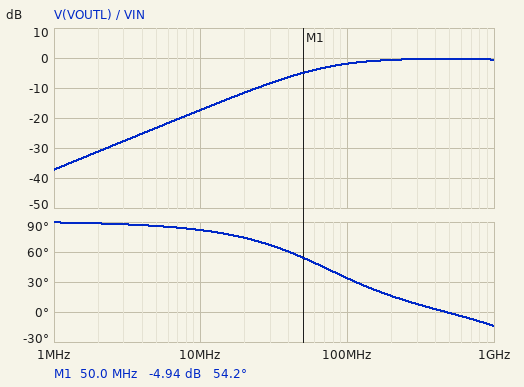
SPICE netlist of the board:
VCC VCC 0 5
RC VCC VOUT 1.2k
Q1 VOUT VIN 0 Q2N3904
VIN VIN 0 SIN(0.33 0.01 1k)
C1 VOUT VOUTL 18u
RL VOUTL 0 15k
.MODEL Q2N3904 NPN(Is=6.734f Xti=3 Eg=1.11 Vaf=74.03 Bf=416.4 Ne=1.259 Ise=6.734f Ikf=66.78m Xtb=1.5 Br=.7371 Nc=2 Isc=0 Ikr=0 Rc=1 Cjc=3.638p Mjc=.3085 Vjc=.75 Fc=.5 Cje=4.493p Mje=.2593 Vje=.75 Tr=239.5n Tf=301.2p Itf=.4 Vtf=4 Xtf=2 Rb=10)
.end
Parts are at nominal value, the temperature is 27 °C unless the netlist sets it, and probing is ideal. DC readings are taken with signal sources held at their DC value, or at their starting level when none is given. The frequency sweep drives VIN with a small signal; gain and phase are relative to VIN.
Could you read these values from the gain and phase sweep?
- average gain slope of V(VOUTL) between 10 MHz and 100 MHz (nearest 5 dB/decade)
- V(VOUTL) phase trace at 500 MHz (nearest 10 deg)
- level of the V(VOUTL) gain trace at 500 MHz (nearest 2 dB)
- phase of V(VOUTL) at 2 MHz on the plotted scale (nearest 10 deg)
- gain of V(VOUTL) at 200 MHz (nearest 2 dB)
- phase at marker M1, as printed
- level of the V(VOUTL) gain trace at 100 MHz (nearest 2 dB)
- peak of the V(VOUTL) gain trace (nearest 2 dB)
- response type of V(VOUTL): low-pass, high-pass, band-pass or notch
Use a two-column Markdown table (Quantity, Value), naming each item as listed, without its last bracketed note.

| Quantity | Value |
|---|---|
| average gain slope of V(VOUTL) between 10 MHz and 100 MHz | 15 dB/decade |
| V(VOUTL) phase trace at 500 MHz | 0 deg |
| level of the V(VOUTL) gain trace at 500 MHz | 0 dB |
| phase of V(VOUTL) at 2 MHz on the plotted scale | 90 deg |
| gain of V(VOUTL) at 200 MHz | 0 dB |
| phase at marker M1, as printed | 54.2 deg |
| level of the V(VOUTL) gain trace at 100 MHz | -2 dB |
| peak of the V(VOUTL) gain trace | 0 dB |
| response type of V(VOUTL): low-pass, high-pass, band-pass or notch | high-pass |
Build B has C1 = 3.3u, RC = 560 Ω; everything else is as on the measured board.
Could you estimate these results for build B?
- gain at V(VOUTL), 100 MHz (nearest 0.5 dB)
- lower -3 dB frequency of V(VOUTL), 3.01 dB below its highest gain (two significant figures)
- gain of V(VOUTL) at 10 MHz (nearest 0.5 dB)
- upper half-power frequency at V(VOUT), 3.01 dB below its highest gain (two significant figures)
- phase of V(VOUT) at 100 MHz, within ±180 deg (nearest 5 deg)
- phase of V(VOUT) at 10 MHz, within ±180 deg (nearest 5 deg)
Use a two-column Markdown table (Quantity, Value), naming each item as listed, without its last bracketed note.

| Quantity | Value |
|---|---|
| gain at V(VOUTL), 100 MHz | -5.0 dB |
| lower -3 dB frequency of V(VOUTL), 3.01 dB below its highest gain | 130 MHz |
| gain of V(VOUTL) at 10 MHz | -23.5 dB |
| upper half-power frequency at V(VOUT), 3.01 dB below its highest gain | 3.4 GHz |
| phase of V(VOUT) at 100 MHz, within ±180 deg | 55 deg |
| phase of V(VOUT) at 10 MHz, within ±180 deg | 85 deg |
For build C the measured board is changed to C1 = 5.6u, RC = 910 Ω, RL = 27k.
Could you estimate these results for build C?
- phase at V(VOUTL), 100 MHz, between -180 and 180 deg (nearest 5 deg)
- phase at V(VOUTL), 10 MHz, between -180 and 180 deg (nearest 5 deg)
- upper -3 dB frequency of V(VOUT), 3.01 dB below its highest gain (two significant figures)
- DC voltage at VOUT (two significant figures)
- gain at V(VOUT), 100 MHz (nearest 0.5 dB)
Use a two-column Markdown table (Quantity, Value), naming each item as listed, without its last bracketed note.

| Quantity | Value |
|---|---|
| phase at V(VOUTL), 100 MHz, between -180 and 180 deg | 40 deg |
| phase at V(VOUTL), 10 MHz, between -180 and 180 deg | 85 deg |
| upper -3 dB frequency of V(VOUT), 3.01 dB below its highest gain | 3.3 GHz |
| DC voltage at VOUT | 5.0 V |
| gain at V(VOUT), 100 MHz | -2.5 dB |
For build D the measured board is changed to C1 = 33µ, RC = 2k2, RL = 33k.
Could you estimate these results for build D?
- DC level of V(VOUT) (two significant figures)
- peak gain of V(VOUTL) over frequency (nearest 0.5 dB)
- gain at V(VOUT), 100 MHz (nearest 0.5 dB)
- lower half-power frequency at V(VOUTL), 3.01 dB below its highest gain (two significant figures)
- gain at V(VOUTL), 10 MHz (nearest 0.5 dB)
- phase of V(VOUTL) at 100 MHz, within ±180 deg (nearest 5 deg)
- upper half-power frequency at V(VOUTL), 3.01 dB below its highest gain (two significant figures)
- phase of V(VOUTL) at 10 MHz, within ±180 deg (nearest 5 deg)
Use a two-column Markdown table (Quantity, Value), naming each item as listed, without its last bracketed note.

| Quantity | Value |
|---|---|
| DC level of V(VOUT) | 5.0 V |
| peak gain of V(VOUTL) over frequency | 0 dB |
| gain at V(VOUT), 100 MHz | -0.5 dB |
| lower half-power frequency at V(VOUTL), 3.01 dB below its highest gain | 38 MHz |
| gain at V(VOUTL), 10 MHz | -12.0 dB |
| phase of V(VOUTL) at 100 MHz, within ±180 deg | 20 deg |
| upper half-power frequency at V(VOUTL), 3.01 dB below its highest gain | 3.1 GHz |
| phase of V(VOUTL) at 10 MHz, within ±180 deg | 75 deg |
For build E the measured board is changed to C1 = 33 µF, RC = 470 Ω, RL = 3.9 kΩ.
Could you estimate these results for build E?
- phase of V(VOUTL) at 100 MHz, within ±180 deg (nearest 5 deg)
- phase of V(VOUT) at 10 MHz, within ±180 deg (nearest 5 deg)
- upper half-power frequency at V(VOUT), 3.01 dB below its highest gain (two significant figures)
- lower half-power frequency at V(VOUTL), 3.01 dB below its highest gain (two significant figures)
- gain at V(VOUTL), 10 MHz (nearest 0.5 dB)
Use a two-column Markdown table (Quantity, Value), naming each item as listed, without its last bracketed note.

| Quantity | Value |
|---|---|
| phase of V(VOUTL) at 100 MHz, within ±180 deg | 60 deg |
| phase of V(VOUT) at 10 MHz, within ±180 deg | 85 deg |
| upper half-power frequency at V(VOUT), 3.01 dB below its highest gain | 3.5 GHz |
| lower half-power frequency at V(VOUTL), 3.01 dB below its highest gain | 170 MHz |
| gain at V(VOUTL), 10 MHz | -25.5 dB |
